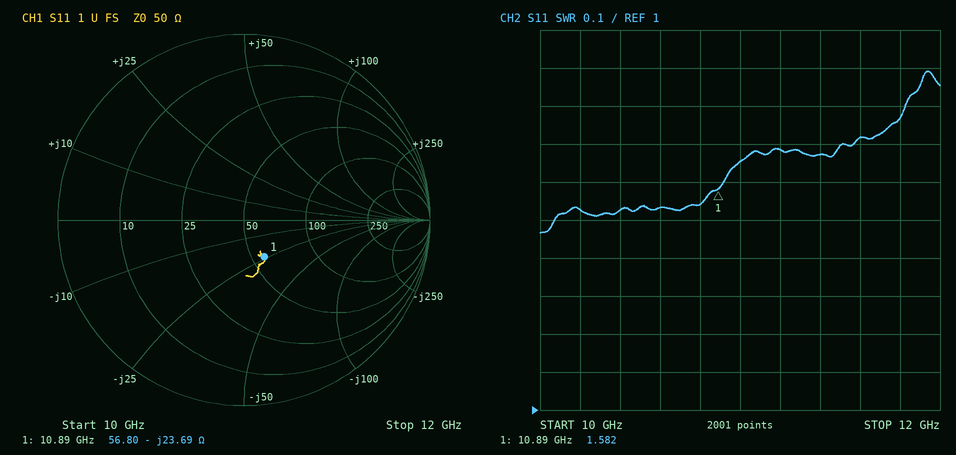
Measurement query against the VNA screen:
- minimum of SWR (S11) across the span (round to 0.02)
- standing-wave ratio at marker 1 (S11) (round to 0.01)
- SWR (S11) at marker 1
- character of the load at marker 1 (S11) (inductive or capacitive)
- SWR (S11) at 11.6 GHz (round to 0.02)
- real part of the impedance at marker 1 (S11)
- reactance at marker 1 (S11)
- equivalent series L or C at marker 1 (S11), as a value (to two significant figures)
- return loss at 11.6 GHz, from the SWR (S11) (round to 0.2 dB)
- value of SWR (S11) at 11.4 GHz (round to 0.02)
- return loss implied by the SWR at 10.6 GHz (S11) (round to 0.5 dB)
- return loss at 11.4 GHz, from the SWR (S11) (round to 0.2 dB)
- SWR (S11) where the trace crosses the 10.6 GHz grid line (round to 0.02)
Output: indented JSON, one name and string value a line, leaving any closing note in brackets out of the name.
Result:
{
  "minimum of SWR (S11) across the span": "1.46",
  "standing-wave ratio at marker 1 (S11)": "1.58",
  "SWR (S11) at marker 1": "1.582",
  "character of the load at marker 1 (S11)": "capacitive",
  "SWR (S11) at 11.6 GHz": "1.72",
  "real part of the impedance at marker 1": "56.80 Ω",
  "reactance at marker 1": "-23.69 Ω",
  "equivalent series L or C at marker 1 (S11), as a value": "620 fF",
  "return loss at 11.6 GHz, from the SWR (S11)": "11.6 dB",
  "value of SWR (S11) at 11.4 GHz": "1.68",
  "return loss implied by the SWR at 10.6 GHz (S11)": "13.5 dB",
  "return loss at 11.4 GHz, from the SWR (S11)": "12.0 dB",
  "SWR (S11) where the trace crosses the 10.6 GHz grid line": "1.54"
}
